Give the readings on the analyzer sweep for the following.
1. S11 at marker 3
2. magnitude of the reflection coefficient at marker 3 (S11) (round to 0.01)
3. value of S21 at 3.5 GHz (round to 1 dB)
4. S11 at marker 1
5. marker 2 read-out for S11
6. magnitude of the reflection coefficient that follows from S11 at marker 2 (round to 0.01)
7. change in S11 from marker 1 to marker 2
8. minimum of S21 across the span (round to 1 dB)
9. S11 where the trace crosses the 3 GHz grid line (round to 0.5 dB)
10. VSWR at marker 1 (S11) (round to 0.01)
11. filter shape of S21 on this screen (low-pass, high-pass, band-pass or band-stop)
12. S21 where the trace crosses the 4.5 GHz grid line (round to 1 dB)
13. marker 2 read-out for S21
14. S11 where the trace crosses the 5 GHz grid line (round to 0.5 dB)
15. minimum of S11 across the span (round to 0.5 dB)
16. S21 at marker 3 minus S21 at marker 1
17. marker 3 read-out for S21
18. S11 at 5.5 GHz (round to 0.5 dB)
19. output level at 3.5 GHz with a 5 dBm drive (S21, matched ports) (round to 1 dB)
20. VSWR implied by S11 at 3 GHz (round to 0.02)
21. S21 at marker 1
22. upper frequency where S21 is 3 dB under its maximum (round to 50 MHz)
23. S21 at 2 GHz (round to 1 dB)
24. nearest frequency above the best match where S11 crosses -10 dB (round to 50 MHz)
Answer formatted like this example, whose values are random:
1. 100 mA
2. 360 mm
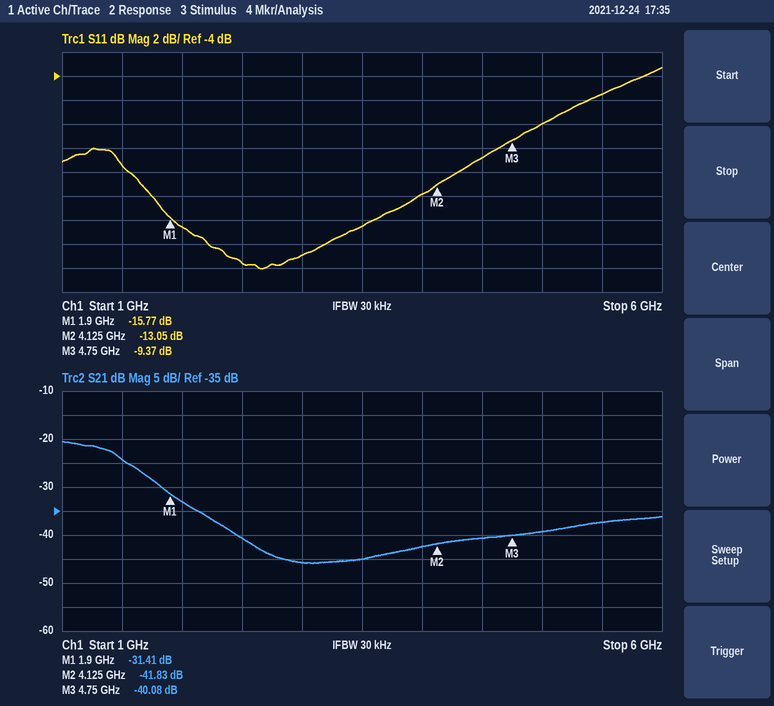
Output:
1. -9.37 dB
2. 0.34
3. -45 dB
4. -15.77 dB
5. -13.05 dB
6. 0.22
7. 2.72 dB
8. -46 dB
9. -19.0 dB
10. 1.39
11. low-pass
12. -41 dB
13. -41.83 dB
14. -8.0 dB
15. -20.0 dB
16. -8.67 dB
17. -40.08 dB
18. -5.5 dB
19. -40 dBm
20. 1.26
21. -31.41 dB
22. 1.45 GHz
23. -33 dB
24. 4.65 GHz
